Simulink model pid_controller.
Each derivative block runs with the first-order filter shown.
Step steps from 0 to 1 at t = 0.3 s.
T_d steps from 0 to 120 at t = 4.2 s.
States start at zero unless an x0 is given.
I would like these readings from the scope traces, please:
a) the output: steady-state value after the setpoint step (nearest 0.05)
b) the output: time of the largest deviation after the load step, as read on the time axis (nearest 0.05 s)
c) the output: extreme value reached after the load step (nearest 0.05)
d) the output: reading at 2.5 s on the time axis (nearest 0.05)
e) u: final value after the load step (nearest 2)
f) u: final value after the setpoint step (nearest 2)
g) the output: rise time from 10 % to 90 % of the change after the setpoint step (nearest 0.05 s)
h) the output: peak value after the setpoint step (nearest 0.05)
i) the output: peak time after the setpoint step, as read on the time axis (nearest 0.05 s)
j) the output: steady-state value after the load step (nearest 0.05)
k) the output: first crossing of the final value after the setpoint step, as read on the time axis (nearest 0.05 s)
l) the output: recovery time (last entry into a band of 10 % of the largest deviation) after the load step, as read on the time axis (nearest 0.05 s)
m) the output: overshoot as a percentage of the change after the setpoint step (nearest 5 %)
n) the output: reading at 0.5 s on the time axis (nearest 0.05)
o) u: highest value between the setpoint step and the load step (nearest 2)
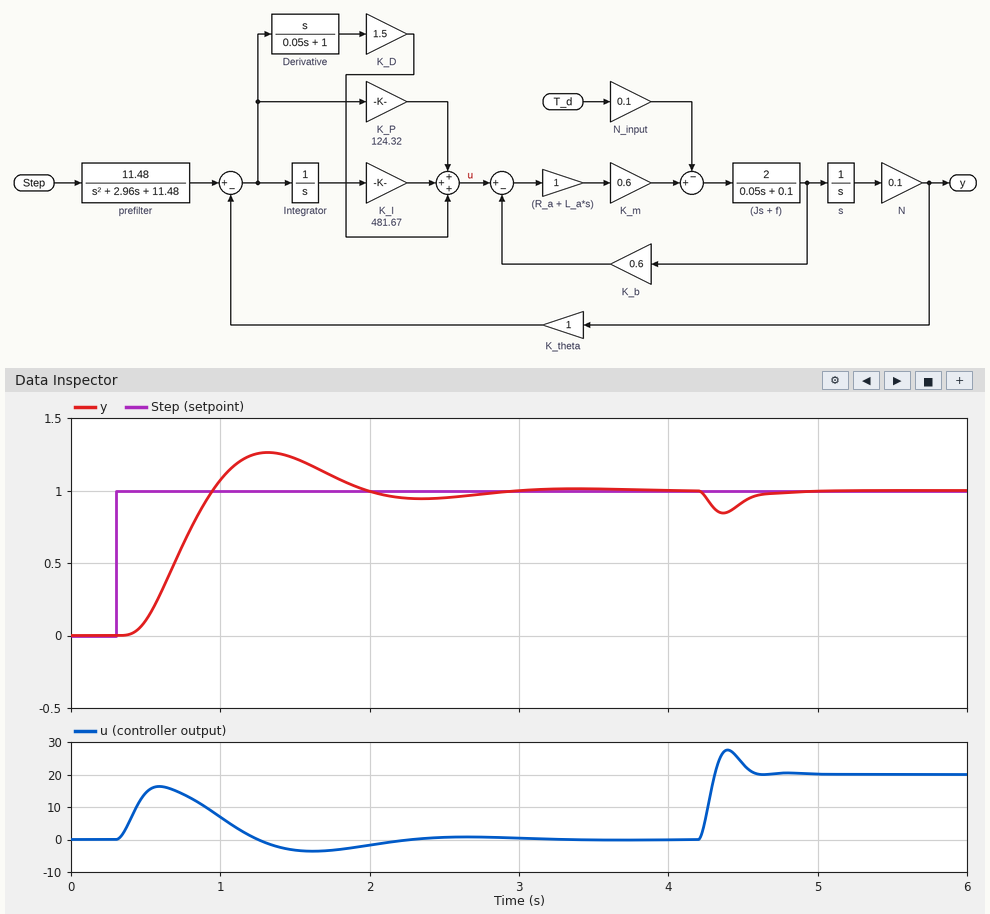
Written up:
1.00
4.35 s
0.85
0.95
20
0
0.40 s
1.25
1.30 s
1.00
0.95 s
4.80 s
25 %
0.10
16
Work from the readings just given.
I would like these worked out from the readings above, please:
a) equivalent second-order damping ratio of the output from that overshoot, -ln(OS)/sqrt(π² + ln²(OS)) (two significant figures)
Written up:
0.40
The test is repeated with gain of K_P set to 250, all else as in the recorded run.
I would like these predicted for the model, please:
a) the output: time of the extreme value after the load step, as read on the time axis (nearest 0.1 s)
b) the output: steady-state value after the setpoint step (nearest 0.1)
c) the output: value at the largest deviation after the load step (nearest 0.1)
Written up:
4.3 s
1.0
0.9
